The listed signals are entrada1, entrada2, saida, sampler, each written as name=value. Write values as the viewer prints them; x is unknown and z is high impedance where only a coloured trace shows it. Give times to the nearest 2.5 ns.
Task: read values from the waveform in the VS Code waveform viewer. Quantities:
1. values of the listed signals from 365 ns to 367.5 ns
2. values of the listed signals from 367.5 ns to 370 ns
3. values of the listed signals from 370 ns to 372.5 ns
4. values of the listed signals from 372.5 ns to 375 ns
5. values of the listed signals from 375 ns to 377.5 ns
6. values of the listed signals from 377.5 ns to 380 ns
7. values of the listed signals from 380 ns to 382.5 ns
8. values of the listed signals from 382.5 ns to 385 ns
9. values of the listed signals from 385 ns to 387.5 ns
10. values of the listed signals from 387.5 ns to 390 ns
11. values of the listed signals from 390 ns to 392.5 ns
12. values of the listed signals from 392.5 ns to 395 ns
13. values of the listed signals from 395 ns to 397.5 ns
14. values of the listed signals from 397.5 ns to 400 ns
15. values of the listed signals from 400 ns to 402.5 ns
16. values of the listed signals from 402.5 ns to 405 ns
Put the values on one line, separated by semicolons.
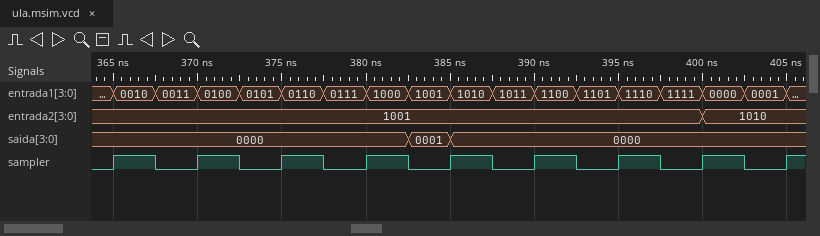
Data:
entrada1=0010, entrada2=1001, saida=0000, sampler=1; entrada1=0011, entrada2=1001, saida=0000, sampler=0; entrada1=0100, entrada2=1001, saida=0000, sampler=1; entrada1=0101, entrada2=1001, saida=0000, sampler=0; entrada1=0110, entrada2=1001, saida=0000, sampler=1; entrada1=0111, entrada2=1001, saida=0000, sampler=0; entrada1=1000, entrada2=1001, saida=0000, sampler=1; entrada1=1001, entrada2=1001, saida=0001, sampler=0; entrada1=1010, entrada2=1001, saida=0000, sampler=1; entrada1=1011, entrada2=1001, saida=0000, sampler=0; entrada1=1100, entrada2=1001, saida=0000, sampler=1; entrada1=1101, entrada2=1001, saida=0000, sampler=0; entrada1=1110, entrada2=1001, saida=0000, sampler=1; entrada1=1111, entrada2=1001, saida=0000, sampler=0; entrada1=0000, entrada2=1010, saida=0000, sampler=1; entrada1=0001, entrada2=1010, saida=0000, sampler=0
